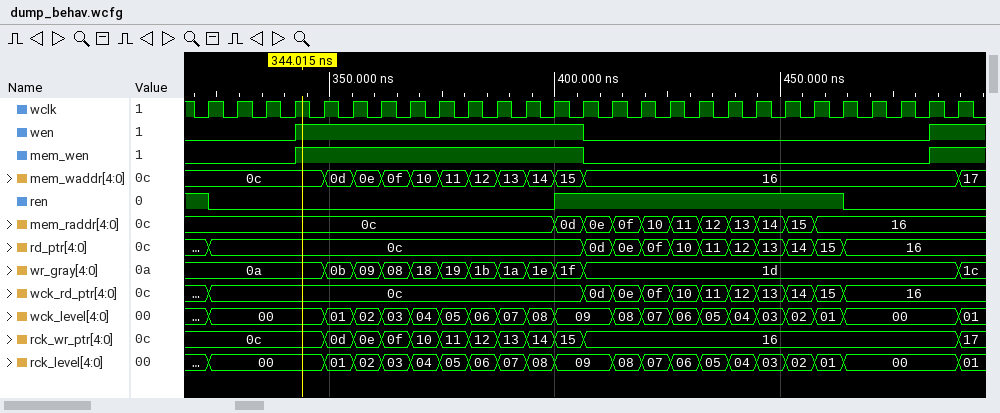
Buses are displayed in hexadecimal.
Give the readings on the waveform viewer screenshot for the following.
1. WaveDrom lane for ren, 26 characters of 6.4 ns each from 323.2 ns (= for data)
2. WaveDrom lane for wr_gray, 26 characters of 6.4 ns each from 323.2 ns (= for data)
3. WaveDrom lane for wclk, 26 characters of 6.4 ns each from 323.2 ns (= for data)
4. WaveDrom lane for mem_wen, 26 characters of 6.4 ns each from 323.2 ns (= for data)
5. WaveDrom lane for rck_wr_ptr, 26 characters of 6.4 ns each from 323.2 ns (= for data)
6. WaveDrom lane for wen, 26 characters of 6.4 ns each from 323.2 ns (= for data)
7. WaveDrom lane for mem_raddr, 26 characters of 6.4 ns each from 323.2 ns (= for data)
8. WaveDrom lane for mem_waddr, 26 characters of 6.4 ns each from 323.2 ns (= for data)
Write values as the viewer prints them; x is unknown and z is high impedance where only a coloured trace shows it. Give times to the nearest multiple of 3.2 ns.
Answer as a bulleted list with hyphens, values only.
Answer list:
- {name: 'ren', wave: '0...........1.........0...'}
- {name: 'wr_gray', wave: '=...==========............', data: '0a 0b 09 08 18 19 1b 1a 1e 1f 1d'}
- {name: 'wclk', wave: 'p.........................'}
- {name: 'mem_wen', wave: '0..1.........0...........1'}
- {name: 'rck_wr_ptr', wave: '=...==========............', data: '0c 0d 0e 0f 10 11 12 13 14 15 16'}
- {name: 'wen', wave: '0..1.........0...........1'}
- {name: 'mem_raddr', wave: '=...........==========....', data: '0c 0d 0e 0f 10 11 12 13 14 15 16'}
- {name: 'mem_waddr', wave: '=...==========............', data: '0c 0d 0e 0f 10 11 12 13 14 15 16'}
